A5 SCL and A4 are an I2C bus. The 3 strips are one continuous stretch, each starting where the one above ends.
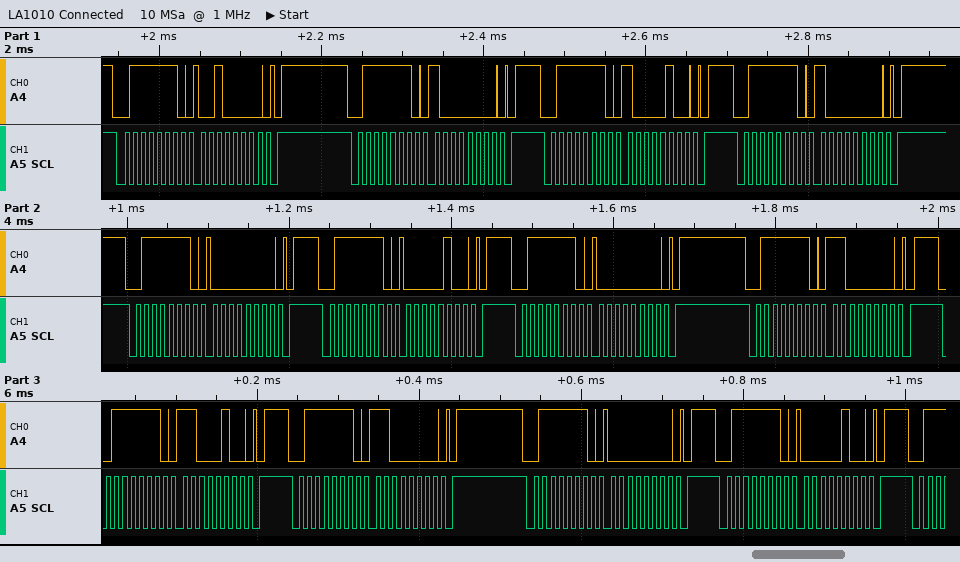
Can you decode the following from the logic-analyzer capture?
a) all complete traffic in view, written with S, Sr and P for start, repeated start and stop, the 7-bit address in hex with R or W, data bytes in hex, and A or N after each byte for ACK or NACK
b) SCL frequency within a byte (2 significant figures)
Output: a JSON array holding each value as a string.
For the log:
["S 3FW A 20 A P S 3FW A 80 A P S 3FW A 84 A P S 3FW A 80 A P S 3FW A 00 A P S 3FW A 04 A P S 3FW A 00 A P S 3FW A C0 A P S 3FW A C4 A P S 3FW A C0 A P S 3FW A 00 A P S 3FW A 04 A P", "100 kHz"]
